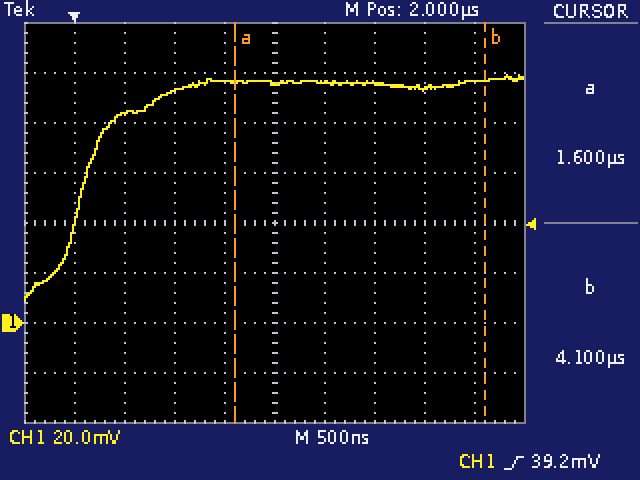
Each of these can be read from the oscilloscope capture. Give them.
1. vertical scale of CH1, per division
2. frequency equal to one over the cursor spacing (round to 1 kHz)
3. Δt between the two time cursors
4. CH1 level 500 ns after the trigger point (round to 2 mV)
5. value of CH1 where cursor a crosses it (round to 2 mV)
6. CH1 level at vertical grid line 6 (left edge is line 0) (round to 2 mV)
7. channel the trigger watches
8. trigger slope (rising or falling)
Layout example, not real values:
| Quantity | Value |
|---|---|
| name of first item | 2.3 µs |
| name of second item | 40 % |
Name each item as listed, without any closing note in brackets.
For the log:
| Quantity | Value |
|---|---|
| vertical scale of CH1, per division | 20 mV |
| frequency equal to one over the cursor spacing | 400 kHz |
| Δt between the two time cursors | 2.50 µs |
| CH1 level 500 ns after the trigger point | 84 mV |
| value of CH1 where cursor a crosses it | 96 mV |
| CH1 level at vertical grid line 6 (left edge is line 0) | 96 mV |
| channel the trigger watches | CH1 |
| trigger slope | rising |
